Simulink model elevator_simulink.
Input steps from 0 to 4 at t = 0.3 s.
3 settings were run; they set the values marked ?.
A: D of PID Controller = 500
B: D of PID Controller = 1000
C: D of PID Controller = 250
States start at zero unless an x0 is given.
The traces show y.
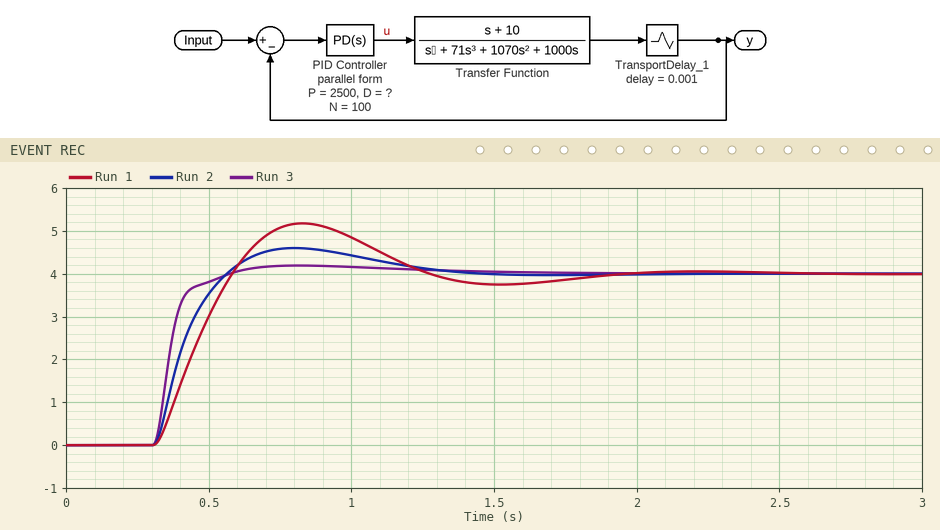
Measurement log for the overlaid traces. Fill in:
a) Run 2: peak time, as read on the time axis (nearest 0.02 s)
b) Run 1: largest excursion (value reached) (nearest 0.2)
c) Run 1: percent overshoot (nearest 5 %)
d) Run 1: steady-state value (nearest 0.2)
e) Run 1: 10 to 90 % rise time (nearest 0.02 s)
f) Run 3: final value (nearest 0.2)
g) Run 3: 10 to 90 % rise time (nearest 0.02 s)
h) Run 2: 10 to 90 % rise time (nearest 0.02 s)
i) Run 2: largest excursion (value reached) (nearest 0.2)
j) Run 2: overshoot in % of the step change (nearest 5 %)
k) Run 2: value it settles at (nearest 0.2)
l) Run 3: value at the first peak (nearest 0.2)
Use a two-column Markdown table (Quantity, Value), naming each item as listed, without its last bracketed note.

| Quantity | Value |
|---|---|
| Run 2: peak time, as read on the time axis | 0.80 s |
| Run 1: largest excursion (value reached) | 5.2 |
| Run 1: percent overshoot | 30 % |
| Run 1: steady-state value | 4.0 |
| Run 1: 10 to 90 % rise time | 0.20 s |
| Run 3: final value | 4.0 |
| Run 3: 10 to 90 % rise time | 0.10 s |
| Run 2: 10 to 90 % rise time | 0.18 s |
| Run 2: largest excursion (value reached) | 4.6 |
| Run 2: overshoot in % of the step change | 15 % |
| Run 2: value it settles at | 4.0 |
| Run 3: value at the first peak | 4.2 |
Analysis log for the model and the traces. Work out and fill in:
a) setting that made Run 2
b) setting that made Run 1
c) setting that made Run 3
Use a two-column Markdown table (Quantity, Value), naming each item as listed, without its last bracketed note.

| Quantity | Value |
|---|---|
| setting that made Run 2 | A |
| setting that made Run 1 | C |
| setting that made Run 3 | B |
